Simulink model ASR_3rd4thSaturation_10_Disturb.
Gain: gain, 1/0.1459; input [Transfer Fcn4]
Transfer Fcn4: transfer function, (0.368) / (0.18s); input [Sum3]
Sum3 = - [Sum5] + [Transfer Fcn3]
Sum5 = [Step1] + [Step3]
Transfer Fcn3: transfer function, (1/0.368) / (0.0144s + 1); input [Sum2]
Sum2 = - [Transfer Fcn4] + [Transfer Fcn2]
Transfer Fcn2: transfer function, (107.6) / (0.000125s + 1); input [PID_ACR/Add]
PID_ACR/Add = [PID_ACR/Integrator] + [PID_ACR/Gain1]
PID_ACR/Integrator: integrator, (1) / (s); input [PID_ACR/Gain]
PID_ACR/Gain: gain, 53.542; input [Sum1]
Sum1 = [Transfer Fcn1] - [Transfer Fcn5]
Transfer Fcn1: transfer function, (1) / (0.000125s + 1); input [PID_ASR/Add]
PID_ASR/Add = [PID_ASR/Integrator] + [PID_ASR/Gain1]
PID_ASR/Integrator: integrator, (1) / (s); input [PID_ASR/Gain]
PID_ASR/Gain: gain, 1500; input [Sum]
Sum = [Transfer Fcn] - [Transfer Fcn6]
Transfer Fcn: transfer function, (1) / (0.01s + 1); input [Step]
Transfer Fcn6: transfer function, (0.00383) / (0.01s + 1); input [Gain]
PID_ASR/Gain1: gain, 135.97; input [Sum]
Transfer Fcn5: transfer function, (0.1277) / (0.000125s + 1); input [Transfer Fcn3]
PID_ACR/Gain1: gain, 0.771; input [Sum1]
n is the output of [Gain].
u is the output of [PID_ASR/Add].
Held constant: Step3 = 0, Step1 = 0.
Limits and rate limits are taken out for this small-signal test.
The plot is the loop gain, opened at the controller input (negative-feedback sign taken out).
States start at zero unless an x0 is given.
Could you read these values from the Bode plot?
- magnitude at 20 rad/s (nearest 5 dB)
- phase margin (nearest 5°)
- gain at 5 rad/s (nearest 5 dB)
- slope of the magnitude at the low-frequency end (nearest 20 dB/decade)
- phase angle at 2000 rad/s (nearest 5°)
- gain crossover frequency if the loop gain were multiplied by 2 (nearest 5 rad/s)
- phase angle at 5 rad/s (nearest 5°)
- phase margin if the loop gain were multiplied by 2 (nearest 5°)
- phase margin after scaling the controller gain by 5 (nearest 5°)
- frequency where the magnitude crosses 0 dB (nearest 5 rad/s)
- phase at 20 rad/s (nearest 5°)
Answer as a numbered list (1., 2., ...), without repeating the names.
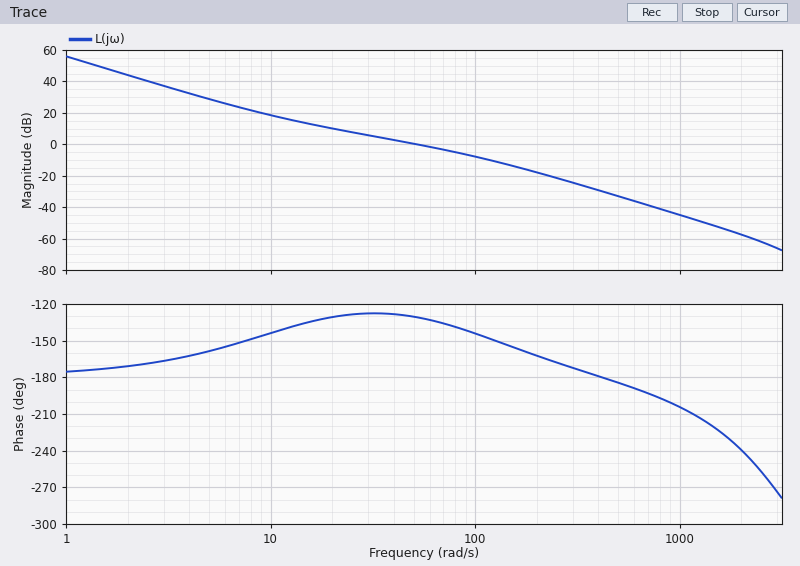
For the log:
1. 10 dB
2. 50°
3. 30 dB
4. -40 dB/decade
5. -240°
6. 85 rad/s
7. -160°
8. 40°
9. 25°
10. 50 rad/s
11. -130°
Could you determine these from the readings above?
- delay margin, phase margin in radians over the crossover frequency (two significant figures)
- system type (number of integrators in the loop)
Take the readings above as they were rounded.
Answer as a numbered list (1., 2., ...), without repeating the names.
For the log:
1. 0.017 s
2. 2
